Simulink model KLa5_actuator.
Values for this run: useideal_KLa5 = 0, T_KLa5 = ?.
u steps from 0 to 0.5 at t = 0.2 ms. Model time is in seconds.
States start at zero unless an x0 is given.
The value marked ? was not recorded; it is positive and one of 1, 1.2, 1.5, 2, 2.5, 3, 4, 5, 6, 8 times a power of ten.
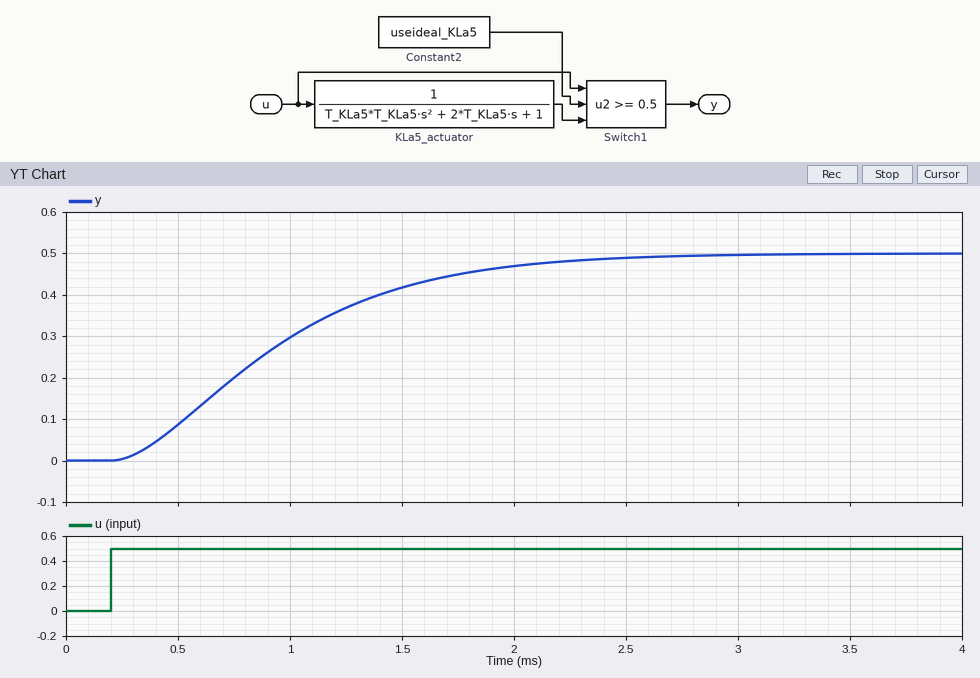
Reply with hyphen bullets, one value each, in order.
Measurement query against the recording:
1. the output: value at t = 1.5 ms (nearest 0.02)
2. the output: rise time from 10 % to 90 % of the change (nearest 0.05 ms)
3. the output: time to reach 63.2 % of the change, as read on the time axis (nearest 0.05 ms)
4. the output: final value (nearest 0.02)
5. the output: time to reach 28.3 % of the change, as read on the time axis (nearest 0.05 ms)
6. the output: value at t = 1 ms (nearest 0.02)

- 0.42
- 1.35 ms
- 1.05 ms
- 0.50
- 0.60 ms
- 0.30
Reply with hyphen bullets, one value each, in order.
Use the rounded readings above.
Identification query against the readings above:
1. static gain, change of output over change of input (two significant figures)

- 1.0
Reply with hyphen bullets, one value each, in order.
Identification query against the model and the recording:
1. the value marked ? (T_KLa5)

- 0.0004
